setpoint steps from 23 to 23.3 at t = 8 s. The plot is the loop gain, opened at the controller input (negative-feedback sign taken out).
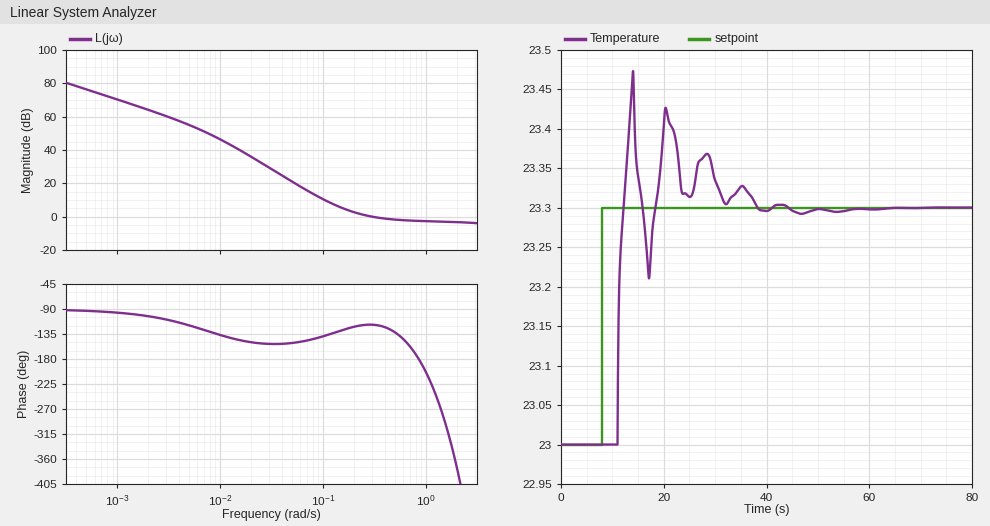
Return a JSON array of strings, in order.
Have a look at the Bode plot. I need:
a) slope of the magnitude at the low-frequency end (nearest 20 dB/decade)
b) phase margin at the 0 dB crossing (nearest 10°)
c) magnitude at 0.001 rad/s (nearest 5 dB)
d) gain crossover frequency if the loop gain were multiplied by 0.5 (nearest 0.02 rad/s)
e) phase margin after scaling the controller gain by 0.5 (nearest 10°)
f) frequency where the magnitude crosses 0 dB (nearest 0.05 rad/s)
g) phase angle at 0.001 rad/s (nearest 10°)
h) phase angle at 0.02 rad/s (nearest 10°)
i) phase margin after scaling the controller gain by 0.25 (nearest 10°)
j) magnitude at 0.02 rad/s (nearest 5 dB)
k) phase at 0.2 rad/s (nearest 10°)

["-20 dB/decade", "60°", "70 dB", "0.14 rad/s", "50°", "0.30 rad/s", "-100°", "-150°", "40°", "35 dB", "-120°"]
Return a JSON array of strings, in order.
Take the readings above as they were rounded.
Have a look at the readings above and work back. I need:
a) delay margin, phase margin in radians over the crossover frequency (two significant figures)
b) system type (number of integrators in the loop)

["3.5 s", "1"]
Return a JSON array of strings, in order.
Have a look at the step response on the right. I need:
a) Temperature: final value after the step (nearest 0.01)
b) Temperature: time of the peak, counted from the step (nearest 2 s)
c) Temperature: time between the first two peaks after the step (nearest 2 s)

["23.30", "6 s", "6 s"]
